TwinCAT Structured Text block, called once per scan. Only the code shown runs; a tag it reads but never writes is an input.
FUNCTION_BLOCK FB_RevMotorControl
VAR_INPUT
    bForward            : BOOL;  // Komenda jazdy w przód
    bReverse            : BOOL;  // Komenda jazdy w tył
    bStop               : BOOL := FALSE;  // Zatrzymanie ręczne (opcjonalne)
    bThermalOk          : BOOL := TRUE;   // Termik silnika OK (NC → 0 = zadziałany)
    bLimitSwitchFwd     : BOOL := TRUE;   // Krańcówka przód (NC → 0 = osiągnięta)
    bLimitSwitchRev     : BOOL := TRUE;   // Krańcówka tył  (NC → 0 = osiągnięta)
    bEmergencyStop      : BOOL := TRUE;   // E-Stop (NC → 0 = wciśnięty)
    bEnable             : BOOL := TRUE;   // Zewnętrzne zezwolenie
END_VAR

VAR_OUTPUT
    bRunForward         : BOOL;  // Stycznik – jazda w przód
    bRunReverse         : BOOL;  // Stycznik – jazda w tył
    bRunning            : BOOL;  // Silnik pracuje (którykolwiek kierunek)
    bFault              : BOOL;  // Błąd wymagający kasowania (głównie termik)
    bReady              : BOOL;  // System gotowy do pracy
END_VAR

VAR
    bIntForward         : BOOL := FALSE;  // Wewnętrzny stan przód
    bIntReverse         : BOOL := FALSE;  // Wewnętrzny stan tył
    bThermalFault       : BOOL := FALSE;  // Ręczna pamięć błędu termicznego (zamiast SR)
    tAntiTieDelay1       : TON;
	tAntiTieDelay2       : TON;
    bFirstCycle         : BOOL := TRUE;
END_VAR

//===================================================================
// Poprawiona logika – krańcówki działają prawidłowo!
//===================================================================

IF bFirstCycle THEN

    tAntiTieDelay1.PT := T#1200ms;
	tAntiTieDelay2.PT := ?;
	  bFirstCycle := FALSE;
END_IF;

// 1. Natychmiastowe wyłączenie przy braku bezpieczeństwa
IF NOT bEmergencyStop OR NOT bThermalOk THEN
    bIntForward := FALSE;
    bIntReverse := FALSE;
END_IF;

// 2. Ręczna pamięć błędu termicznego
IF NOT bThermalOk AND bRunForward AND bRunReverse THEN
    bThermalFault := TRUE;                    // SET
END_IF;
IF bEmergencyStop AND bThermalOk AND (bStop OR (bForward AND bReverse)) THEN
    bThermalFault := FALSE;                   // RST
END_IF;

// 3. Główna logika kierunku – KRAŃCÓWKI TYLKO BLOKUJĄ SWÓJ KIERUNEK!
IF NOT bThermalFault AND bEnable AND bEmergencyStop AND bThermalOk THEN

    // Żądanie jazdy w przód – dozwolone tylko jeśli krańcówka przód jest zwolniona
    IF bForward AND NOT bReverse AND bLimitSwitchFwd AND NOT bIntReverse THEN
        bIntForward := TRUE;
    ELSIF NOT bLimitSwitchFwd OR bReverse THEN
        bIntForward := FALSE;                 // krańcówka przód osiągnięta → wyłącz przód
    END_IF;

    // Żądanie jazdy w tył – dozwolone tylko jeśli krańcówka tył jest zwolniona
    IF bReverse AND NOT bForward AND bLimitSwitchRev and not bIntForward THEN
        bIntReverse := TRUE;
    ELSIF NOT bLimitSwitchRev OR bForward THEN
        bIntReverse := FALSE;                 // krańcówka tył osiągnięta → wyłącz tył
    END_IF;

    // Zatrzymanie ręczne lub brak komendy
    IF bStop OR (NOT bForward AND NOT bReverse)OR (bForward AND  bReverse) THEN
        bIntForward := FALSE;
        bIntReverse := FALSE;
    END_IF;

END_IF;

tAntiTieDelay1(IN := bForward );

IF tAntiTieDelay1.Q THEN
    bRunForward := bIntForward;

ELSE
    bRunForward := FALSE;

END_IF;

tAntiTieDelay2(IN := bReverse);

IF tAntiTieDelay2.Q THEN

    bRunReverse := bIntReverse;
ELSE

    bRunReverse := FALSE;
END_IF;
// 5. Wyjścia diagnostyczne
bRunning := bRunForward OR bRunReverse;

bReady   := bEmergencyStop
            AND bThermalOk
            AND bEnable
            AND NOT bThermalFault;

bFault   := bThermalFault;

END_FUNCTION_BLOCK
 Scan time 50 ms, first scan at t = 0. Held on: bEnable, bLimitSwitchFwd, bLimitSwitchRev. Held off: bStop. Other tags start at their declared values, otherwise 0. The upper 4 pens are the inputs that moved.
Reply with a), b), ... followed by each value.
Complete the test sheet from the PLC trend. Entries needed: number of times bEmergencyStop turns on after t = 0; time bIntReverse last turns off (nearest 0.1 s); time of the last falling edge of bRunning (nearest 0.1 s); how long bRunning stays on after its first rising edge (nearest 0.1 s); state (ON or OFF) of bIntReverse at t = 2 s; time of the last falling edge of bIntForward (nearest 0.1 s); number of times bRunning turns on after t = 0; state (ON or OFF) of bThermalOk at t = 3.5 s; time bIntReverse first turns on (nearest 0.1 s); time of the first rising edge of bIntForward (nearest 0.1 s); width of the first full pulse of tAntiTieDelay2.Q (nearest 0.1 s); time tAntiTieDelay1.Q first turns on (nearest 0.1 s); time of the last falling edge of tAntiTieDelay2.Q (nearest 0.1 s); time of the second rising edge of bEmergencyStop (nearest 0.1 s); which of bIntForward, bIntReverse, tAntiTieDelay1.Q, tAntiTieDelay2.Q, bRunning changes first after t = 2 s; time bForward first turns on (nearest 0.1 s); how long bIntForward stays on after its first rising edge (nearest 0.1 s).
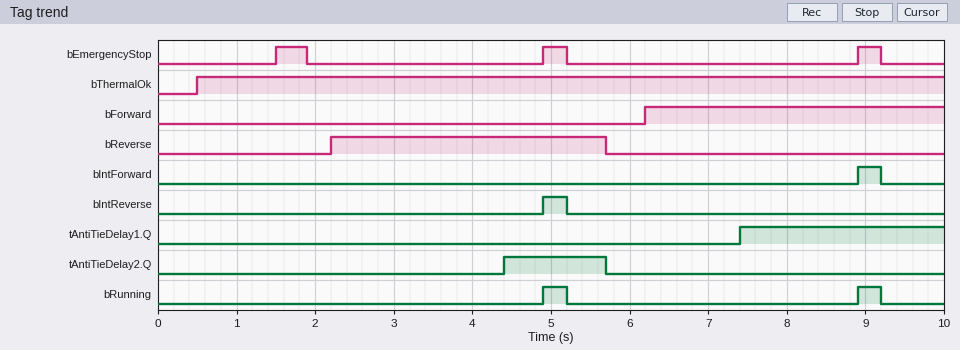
a) 3
b) 5.2 s
c) 9.2 s
d) 0.3 s
e) OFF
f) 9.2 s
g) 2
h) ON
i) 4.9 s
j) 8.9 s
k) 1.3 s
l) 7.4 s
m) 5.7 s
n) 4.9 s
o) tAntiTieDelay2.Q
p) 6.2 s
q) 0.3 s
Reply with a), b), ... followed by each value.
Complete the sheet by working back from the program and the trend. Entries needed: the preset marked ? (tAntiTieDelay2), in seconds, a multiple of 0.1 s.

a) 2.2 s
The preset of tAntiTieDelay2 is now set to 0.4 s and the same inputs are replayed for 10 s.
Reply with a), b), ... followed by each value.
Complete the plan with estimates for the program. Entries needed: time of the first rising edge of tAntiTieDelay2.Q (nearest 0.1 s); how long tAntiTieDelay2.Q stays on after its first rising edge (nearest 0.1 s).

a) 2.6 s
b) 3.1 s
